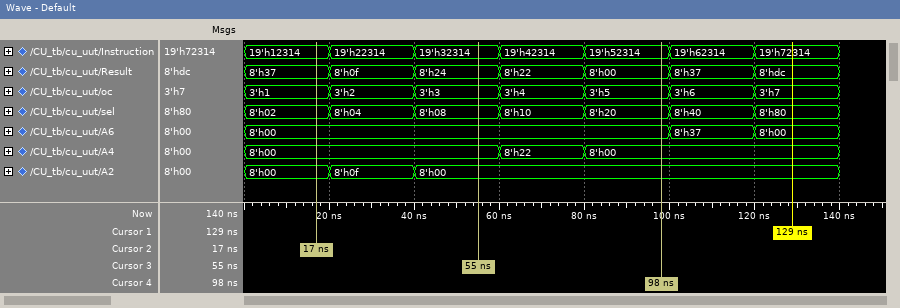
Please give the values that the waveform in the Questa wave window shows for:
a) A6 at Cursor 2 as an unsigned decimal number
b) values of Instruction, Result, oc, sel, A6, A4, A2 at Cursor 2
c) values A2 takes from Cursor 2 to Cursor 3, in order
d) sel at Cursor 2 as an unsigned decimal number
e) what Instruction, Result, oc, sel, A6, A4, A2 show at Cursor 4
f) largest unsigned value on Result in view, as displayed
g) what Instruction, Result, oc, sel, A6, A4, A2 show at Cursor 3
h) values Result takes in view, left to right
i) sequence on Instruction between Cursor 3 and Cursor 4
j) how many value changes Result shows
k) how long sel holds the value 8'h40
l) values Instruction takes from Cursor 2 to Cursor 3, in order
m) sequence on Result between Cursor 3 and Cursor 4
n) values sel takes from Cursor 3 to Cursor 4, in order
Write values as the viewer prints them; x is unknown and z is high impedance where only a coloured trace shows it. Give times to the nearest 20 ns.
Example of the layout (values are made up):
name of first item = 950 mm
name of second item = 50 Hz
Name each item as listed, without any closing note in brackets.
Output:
A6 at Cursor 2 as an unsigned decimal number = 0
values of Instruction, Result, oc, sel, A6, A4, A2 at Cursor 2 = Instruction=19'h12314, Result=8'h37, oc=3'h1, sel=8'h02, A6=8'h00, A4=8'h00, A2=8'h00
values A2 takes from Cursor 2 to Cursor 3, in order = 8'h00, 8'h0f, 8'h00
sel at Cursor 2 as an unsigned decimal number = 2
what Instruction, Result, oc, sel, A6, A4, A2 show at Cursor 4 = Instruction=19'h52314, Result=8'h00, oc=3'h5, sel=8'h20, A6=8'h00, A4=8'h00, A2=8'h00
largest unsigned value on Result in view, as displayed = 8'hdc
what Instruction, Result, oc, sel, A6, A4, A2 show at Cursor 3 = Instruction=19'h32314, Result=8'h24, oc=3'h3, sel=8'h08, A6=8'h00, A4=8'h00, A2=8'h00
values Result takes in view, left to right = 8'h37, 8'h0f, 8'h24, 8'h22, 8'h00, 8'h37, 8'hdc
sequence on Instruction between Cursor 3 and Cursor 4 = 19'h32314, 19'h42314, 19'h52314
how many value changes Result shows = 6
how long sel holds the value 8'h40 = 20 ns
values Instruction takes from Cursor 2 to Cursor 3, in order = 19'h12314, 19'h22314, 19'h32314
sequence on Result between Cursor 3 and Cursor 4 = 8'h24, 8'h22, 8'h00
values sel takes from Cursor 3 to Cursor 4, in order = 8'h08, 8'h10, 8'h20
